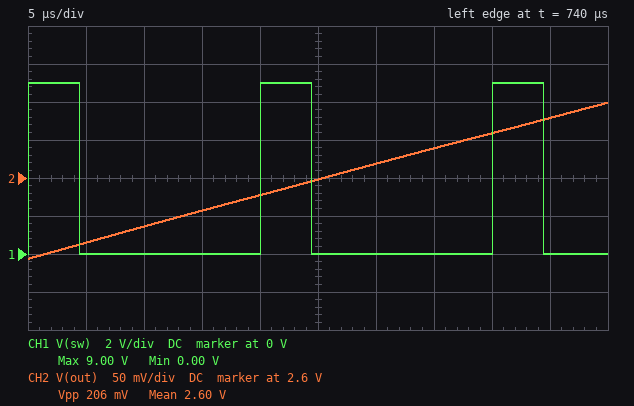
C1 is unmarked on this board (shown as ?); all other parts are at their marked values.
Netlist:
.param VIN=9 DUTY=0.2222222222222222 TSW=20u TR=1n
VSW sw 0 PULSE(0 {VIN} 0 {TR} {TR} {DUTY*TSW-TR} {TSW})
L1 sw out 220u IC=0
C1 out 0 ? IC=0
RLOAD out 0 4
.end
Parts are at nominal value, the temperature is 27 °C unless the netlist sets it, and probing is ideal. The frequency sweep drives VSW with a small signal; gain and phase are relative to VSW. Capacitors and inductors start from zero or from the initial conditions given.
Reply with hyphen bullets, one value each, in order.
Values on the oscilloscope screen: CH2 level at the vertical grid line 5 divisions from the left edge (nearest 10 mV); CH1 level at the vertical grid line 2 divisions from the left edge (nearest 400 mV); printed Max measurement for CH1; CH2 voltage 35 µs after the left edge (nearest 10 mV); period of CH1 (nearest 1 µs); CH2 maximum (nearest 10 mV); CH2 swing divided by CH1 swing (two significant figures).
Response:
- 2.60 V
- 0 V
- 9.00 V
- 2.64 V
- 20 µs
- 2.70 V
- 0.023
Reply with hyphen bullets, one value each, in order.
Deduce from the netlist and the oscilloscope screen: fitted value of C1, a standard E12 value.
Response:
- 680 µF
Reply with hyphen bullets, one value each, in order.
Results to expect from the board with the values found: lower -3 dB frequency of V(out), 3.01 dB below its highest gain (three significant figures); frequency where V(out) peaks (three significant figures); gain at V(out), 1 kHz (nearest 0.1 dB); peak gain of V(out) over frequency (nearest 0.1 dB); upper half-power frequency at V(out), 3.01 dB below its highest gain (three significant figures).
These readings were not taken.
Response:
- 379 Hz
- 409 Hz
- -13.8 dB
- 17.0 dB
- 438 Hz
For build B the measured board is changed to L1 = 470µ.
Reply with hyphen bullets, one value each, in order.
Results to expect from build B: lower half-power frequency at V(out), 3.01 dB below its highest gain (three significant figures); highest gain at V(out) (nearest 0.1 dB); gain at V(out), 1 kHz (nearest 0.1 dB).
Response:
- 247 Hz
- 13.7 dB
- -21.3 dB
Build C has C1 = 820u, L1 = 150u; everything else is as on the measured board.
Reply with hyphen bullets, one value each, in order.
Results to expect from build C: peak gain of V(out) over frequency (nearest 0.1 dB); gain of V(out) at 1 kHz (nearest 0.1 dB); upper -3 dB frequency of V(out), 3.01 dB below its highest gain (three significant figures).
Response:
- 19.4 dB
- -11.7 dB
- 476 Hz
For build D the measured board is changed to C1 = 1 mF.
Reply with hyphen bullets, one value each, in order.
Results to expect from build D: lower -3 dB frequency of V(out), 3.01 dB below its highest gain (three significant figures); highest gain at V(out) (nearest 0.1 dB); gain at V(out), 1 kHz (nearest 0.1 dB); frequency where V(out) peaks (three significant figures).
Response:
- 318 Hz
- 18.6 dB
- -17.7 dB
- 338 Hz
